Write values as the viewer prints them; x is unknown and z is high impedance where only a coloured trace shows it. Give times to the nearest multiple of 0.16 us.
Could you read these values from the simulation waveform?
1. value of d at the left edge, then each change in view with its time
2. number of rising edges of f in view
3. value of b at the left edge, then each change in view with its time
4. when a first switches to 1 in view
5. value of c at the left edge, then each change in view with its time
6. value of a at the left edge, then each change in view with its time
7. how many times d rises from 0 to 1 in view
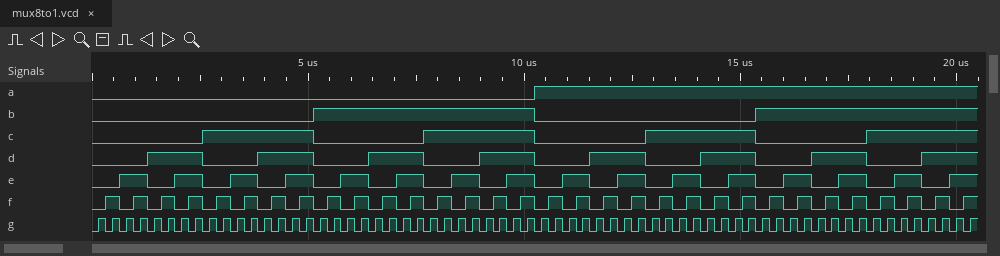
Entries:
0, 1 at 1.28 us, 0 at 2.56 us, 1 at 3.84 us, 0 at 5.12 us, 1 at 6.4 us, 0 at 7.68 us, 1 at 8.96 us, 0 at 10.24 us, 1 at 11.52 us, 0 at 12.8 us, 1 at 14.08 us, 0 at 15.36 us, 1 at 16.64 us, 0 at 17.92 us, 1 at 19.2 us
32
0, 1 at 5.12 us, 0 at 10.24 us, 1 at 15.36 us
10.24 us
0, 1 at 2.56 us, 0 at 5.12 us, 1 at 7.68 us, 0 at 10.24 us, 1 at 12.8 us, 0 at 15.36 us, 1 at 17.92 us
0, 1 at 10.24 us
8
